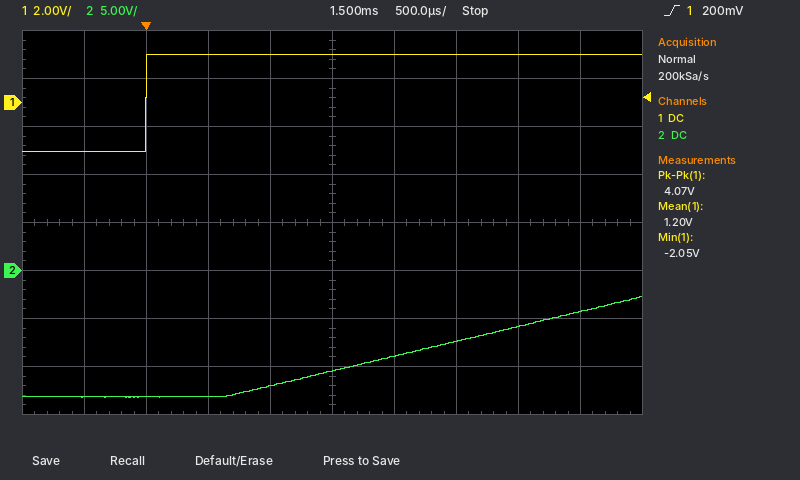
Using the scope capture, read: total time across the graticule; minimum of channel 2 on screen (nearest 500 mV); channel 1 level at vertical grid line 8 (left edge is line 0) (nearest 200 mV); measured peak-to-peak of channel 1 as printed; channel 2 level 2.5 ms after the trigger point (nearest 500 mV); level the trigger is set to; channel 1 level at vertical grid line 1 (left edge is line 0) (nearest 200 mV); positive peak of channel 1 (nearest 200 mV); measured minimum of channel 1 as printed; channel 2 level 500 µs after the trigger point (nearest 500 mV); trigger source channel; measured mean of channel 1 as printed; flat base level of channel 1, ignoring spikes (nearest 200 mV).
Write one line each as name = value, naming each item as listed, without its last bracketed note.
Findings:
total time across the graticule = 5 ms
minimum of channel 2 on screen = -13.0 V
channel 1 level at vertical grid line 8 (left edge is line 0) = 2.0 V
measured peak-to-peak of channel 1 as printed = 4.07 V
channel 2 level 2.5 ms after the trigger point = -7.5 V
level the trigger is set to = 200 mV
channel 1 level at vertical grid line 1 (left edge is line 0) = -2.0 V
positive peak of channel 1 = 2.0 V
measured minimum of channel 1 as printed = -2.05 V
channel 2 level 500 µs after the trigger point = -13.0 V
trigger source channel = channel 1
measured mean of channel 1 as printed = 1.20 V
flat base level of channel 1, ignoring spikes = -2.0 V
